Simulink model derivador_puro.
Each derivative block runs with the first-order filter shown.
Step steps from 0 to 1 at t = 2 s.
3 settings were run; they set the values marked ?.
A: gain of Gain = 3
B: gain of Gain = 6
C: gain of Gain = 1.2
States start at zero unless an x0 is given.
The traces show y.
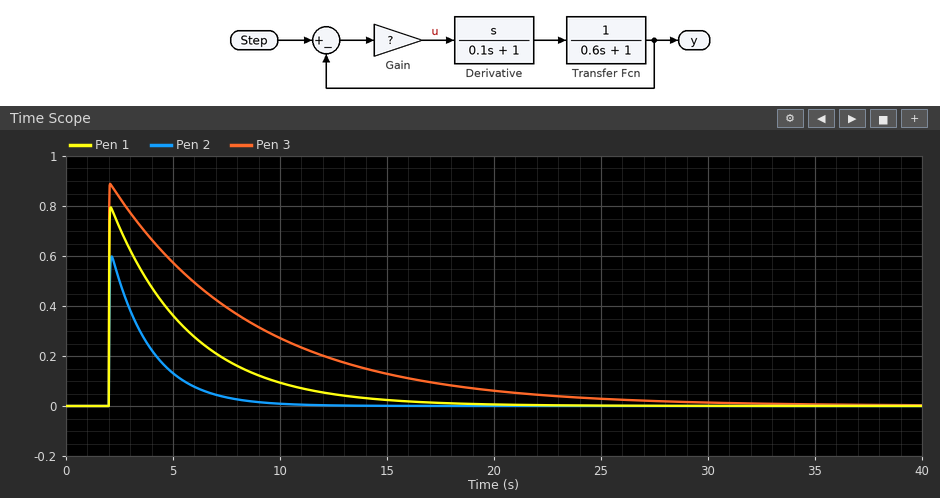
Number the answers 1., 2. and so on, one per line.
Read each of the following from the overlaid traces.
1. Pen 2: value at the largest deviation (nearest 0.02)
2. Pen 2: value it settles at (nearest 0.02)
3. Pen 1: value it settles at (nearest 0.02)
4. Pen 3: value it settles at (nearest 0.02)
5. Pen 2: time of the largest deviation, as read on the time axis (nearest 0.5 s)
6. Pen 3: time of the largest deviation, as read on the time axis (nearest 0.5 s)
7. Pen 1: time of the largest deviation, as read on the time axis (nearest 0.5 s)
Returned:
1. 0.60
2. 0.00
3. 0.00
4. 0.00
5. 2.0 s
6. 2.0 s
7. 2.0 s
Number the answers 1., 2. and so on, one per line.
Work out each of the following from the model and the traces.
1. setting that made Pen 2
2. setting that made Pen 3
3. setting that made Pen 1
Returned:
1. C
2. B
3. A
